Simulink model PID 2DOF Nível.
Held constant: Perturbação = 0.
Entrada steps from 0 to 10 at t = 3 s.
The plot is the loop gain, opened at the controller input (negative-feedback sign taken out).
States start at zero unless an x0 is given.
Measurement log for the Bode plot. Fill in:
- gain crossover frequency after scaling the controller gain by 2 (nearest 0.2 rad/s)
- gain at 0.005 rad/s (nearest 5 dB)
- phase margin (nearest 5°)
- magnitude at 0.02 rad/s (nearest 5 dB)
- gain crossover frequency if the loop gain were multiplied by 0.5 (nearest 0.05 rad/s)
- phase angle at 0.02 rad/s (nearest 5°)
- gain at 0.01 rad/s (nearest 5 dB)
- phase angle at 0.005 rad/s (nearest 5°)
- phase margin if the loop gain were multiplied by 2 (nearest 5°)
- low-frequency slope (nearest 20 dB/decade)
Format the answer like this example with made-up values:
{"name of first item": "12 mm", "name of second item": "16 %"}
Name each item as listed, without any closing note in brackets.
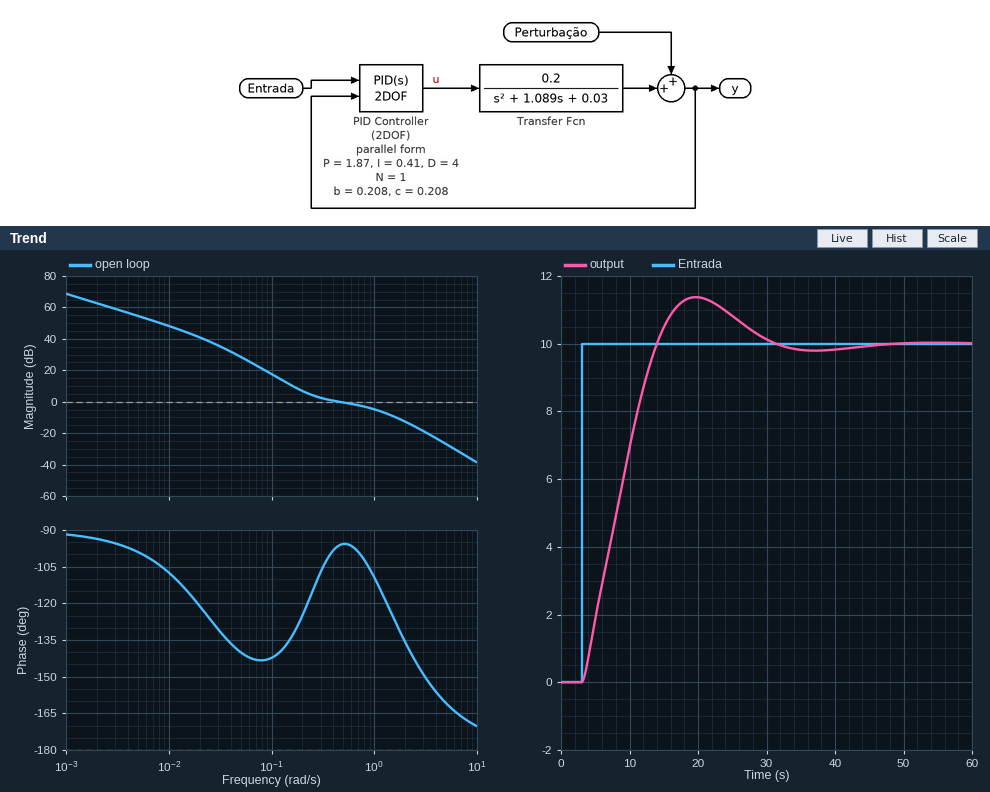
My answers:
{"gain crossover frequency after scaling the controller gain by 2": "1.2 rad/s", "gain at 0.005 rad/s": "55 dB", "phase margin": "85°", "magnitude at 0.02 rad/s": "40 dB", "gain crossover frequency if the loop gain were multiplied by 0.5": "0.20 rad/s", "phase angle at 0.02 rad/s": "-120°", "gain at 0.01 rad/s": "50 dB", "phase angle at 0.005 rad/s": "-100°", "phase margin if the loop gain were multiplied by 2": "65°", "low-frequency slope": "-20 dB/decade"}
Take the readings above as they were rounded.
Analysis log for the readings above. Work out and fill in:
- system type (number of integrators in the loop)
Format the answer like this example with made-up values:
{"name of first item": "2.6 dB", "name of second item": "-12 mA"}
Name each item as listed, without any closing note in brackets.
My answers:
{"system type": "1"}
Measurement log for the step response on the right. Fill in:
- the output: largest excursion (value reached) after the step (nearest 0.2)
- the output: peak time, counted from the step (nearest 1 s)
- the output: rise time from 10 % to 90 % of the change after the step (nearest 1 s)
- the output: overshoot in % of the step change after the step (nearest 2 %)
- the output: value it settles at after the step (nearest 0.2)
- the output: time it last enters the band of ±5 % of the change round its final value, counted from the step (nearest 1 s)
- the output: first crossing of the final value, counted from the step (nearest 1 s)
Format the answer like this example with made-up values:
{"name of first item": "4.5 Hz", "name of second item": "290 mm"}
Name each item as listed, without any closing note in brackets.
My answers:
{"the output: largest excursion (value reached) after the step": "11.4", "the output: peak time, counted from the step": "17 s", "the output: rise time from 10 % to 90 % of the change after the step": "8 s", "the output: overshoot in % of the step change after the step": "14 %", "the output: value it settles at after the step": "10.0", "the output: time it last enters the band of ±5 % of the change round its final value, counted from the step": "24 s", "the output: first crossing of the final value, counted from the step": "11 s"}
